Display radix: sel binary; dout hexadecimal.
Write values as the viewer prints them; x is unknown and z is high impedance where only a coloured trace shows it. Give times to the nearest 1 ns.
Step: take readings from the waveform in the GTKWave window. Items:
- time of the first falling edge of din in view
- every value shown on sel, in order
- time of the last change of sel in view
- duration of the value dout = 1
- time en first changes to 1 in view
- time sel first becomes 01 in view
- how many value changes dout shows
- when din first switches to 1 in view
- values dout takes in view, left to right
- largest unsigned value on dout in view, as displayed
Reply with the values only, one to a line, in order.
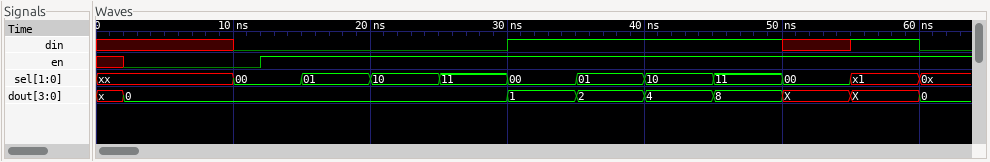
60 ns
xx, 00, 01, 10, 11, 00, 01, 10, 11, 00, x1, 0x
60 ns
5 ns
12 ns
15 ns
8
30 ns
x, 0, 1, 2, 4, 8, X, X, 0
8
